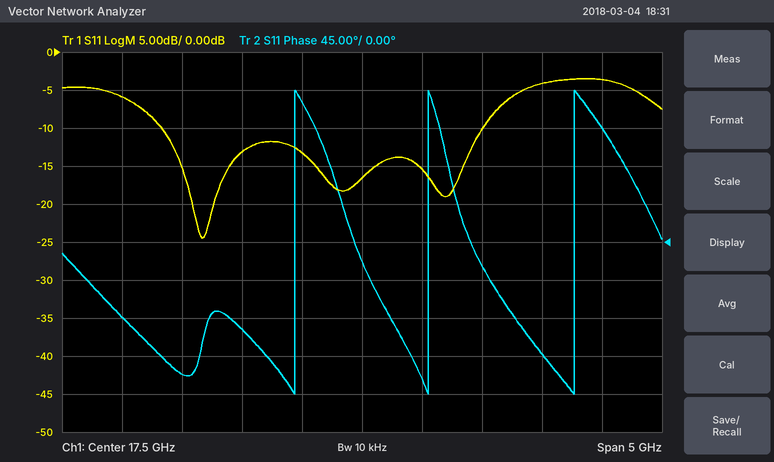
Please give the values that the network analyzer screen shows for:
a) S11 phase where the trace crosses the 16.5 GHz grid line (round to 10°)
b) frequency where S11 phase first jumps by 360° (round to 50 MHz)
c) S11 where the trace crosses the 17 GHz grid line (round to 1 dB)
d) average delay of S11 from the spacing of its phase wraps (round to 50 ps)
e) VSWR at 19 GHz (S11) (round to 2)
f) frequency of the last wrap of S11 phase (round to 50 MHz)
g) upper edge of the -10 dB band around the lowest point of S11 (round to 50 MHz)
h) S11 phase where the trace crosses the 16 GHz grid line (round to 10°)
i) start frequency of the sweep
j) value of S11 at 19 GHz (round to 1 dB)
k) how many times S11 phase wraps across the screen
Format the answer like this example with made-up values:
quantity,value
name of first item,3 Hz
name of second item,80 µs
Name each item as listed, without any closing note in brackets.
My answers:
quantity,value
S11 phase where the trace crosses the 16.5 GHz grid line,-100°
frequency where S11 phase first jumps by 360°,16.95 GHz
S11 where the trace crosses the 17 GHz grid line,-13 dB
average delay of S11 from the spacing of its phase wraps,850 ps
VSWR at 19 GHz (S11),4
frequency of the last wrap of S11 phase,19.25 GHz
upper edge of the -10 dB band around the lowest point of S11,18.50 GHz
S11 phase where the trace crosses the 16 GHz grid line,-160°
start frequency of the sweep,15 GHz
value of S11 at 19 GHz,-4 dB
how many times S11 phase wraps across the screen,3
